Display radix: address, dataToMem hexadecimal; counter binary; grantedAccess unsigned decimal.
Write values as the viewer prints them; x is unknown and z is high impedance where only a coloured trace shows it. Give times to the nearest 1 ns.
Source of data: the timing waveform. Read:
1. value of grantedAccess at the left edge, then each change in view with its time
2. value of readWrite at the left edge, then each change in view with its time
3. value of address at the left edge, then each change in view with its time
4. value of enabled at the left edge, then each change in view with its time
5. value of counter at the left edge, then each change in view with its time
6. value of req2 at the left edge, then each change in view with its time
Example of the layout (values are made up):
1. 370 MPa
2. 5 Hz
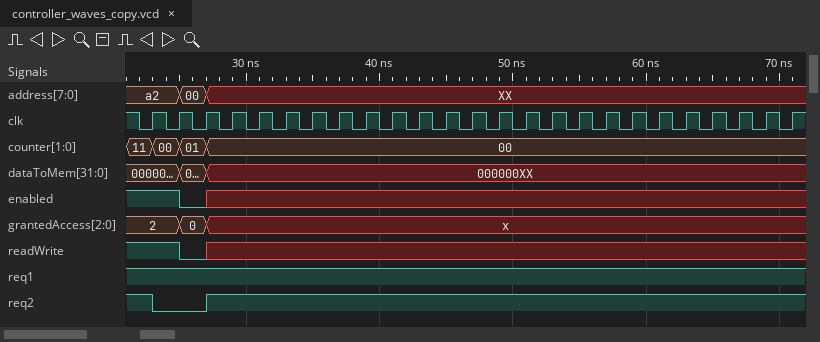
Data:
1. 2, 0 at 25 ns, x at 27 ns
2. 1, 0 at 25 ns, x at 27 ns
3. a2, 00 at 25 ns, XX at 27 ns
4. 1, 0 at 25 ns, x at 27 ns
5. 11, 00 at 23 ns, 01 at 25 ns, 00 at 27 ns
6. 1, 0 at 23 ns, 1 at 27 ns
